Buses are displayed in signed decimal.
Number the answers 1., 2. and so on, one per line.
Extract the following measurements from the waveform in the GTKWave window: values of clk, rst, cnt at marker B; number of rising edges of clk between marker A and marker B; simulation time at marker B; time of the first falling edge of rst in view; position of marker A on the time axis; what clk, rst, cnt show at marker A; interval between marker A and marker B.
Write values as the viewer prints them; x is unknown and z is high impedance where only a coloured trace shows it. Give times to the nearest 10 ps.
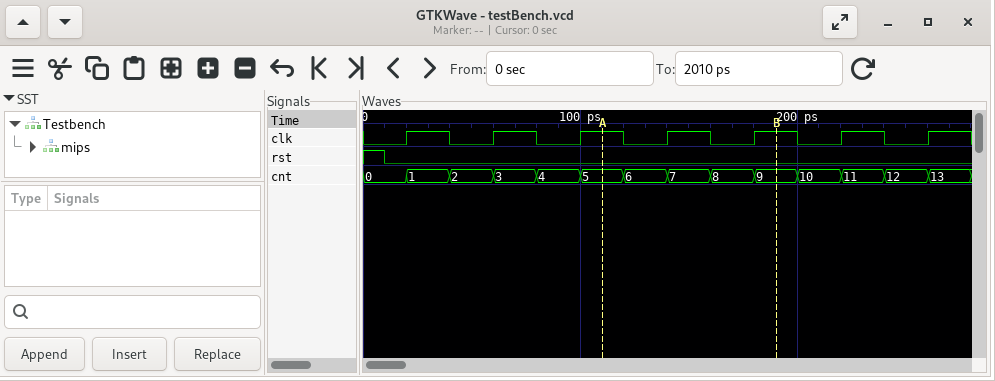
1. clk=1, rst=0, cnt=9
2. 2
3. 190 ps
4. 10 ps
5. 110 ps
6. clk=1, rst=0, cnt=5
7. 80 ps
